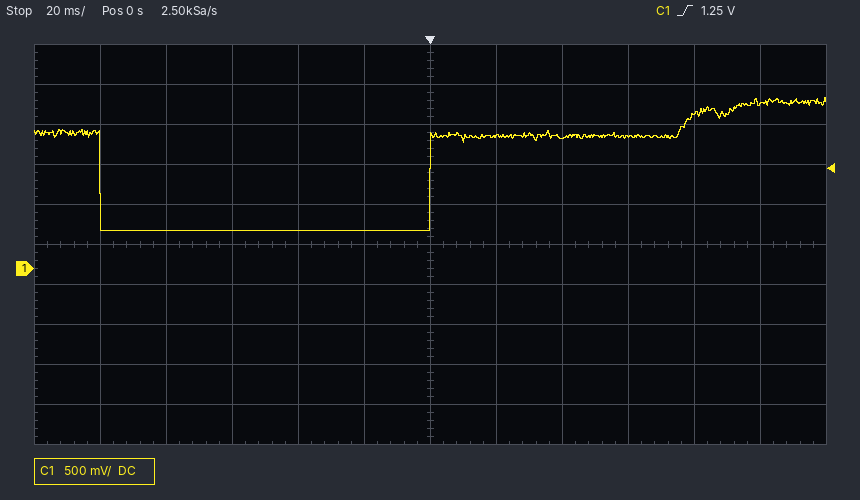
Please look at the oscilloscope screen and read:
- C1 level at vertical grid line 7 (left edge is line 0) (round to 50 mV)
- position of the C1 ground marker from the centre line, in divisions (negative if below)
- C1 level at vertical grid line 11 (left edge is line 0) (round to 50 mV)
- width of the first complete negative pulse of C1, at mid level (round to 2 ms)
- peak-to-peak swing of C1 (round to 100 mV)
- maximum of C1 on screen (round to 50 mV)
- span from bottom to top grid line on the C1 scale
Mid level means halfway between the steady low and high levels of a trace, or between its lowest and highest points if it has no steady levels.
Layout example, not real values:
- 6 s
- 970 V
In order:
- 1.65 V
- -0.6 div
- 2.05 V
- 100 ms
- 1.70 V
- 2.15 V
- 5 V
